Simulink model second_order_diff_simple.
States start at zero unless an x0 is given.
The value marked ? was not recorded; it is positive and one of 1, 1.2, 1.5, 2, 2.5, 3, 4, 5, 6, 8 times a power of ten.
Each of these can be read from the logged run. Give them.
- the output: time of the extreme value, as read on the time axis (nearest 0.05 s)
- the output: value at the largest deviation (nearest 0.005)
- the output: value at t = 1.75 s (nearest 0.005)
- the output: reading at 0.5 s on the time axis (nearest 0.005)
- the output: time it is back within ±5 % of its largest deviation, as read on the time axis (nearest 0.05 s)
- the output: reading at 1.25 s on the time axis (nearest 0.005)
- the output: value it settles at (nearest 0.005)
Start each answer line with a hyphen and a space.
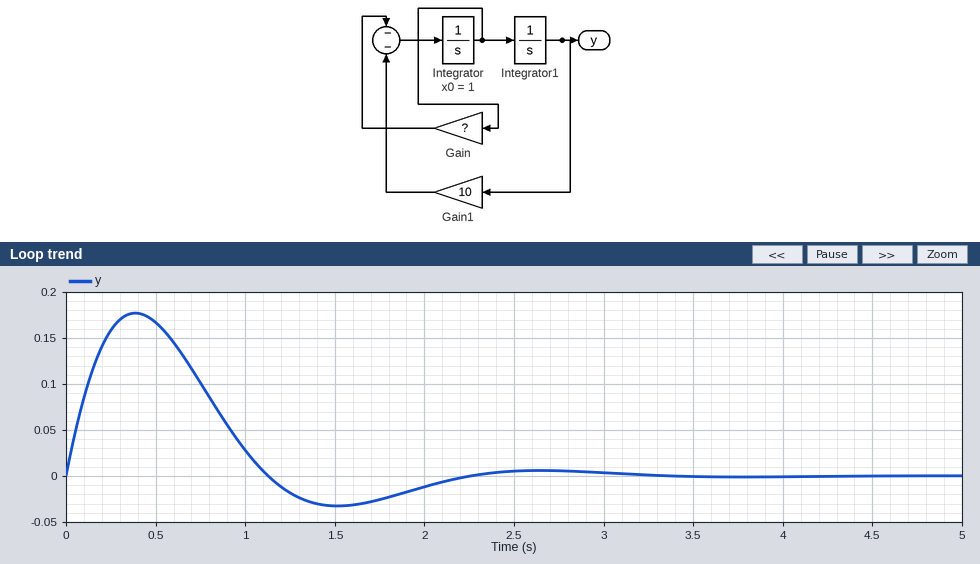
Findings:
- 0.40 s
- 0.175
- -0.025
- 0.165
- 2.05 s
- -0.020
- 0.000
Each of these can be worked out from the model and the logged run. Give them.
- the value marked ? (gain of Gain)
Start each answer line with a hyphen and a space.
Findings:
- 3
